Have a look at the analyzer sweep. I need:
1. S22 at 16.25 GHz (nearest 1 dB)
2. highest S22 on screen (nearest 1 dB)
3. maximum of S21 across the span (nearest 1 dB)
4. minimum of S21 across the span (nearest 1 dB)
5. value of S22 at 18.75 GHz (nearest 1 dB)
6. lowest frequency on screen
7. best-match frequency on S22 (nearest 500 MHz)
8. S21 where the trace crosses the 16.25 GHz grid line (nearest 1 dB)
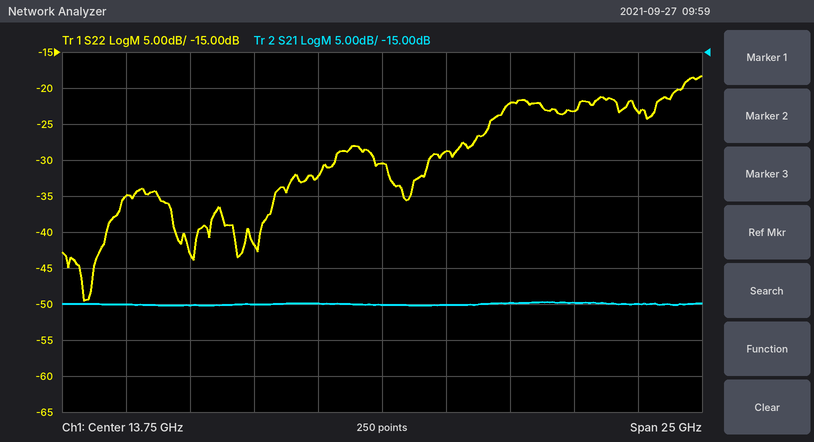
-29 dB
-18 dB
-50 dB
-50 dB
-22 dB
1.25 GHz
2.0 GHz
-50 dB
